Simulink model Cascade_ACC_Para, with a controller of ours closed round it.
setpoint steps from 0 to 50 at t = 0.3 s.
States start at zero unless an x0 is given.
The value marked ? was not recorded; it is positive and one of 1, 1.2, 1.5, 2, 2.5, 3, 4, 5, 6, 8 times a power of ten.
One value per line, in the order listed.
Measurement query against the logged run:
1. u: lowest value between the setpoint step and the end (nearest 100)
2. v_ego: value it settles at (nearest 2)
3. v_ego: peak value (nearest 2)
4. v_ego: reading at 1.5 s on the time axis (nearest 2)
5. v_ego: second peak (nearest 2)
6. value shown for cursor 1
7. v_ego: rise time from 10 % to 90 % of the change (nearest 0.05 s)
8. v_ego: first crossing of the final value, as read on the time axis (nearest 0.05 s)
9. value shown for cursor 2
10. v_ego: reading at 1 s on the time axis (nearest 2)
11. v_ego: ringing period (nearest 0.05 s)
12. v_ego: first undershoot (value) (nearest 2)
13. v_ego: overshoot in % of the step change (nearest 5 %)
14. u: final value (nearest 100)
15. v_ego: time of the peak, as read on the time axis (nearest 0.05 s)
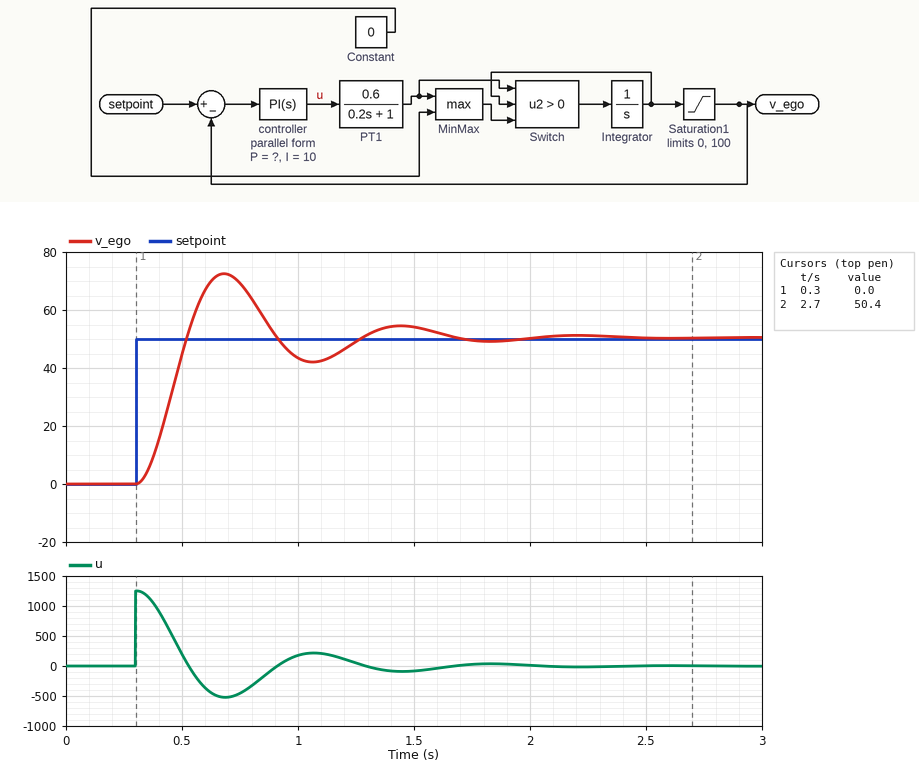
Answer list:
-500
50
72
54
54
0.0
0.15 s
0.50 s
50.4
44
0.75 s
42
45 %
0
0.70 s
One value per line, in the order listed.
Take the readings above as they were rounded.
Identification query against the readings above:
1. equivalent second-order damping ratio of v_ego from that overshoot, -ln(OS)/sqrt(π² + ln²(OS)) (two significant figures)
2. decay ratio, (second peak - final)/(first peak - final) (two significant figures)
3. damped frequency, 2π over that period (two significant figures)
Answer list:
0.25
0.18
8.4 rad/s
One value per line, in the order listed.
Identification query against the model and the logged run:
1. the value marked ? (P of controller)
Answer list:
25
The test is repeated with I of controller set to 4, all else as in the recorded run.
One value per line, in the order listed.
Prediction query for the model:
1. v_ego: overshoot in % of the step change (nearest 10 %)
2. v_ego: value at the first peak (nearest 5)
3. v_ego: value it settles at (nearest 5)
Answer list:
40 %
70
50
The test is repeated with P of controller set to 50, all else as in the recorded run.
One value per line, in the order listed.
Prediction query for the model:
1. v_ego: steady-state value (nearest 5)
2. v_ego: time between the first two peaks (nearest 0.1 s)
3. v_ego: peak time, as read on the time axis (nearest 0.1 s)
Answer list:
50
0.5 s
0.6 s
